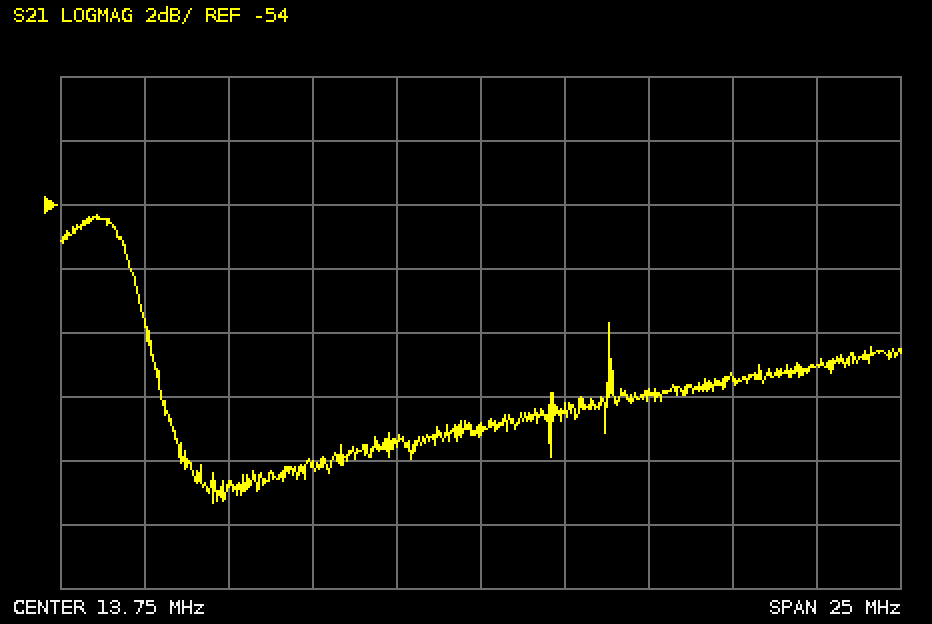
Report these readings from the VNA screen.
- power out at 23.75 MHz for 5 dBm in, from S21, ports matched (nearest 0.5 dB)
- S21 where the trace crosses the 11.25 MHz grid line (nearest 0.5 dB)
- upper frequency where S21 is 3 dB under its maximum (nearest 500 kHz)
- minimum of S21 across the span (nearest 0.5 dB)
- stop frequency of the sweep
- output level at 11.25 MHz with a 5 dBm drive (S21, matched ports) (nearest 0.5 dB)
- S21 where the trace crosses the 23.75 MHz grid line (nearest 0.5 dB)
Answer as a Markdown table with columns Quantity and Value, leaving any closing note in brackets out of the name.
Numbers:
| Quantity | Value |
|---|---|
| power out at 23.75 MHz for 5 dBm in, from S21, ports matched | -54.0 dBm |
| S21 where the trace crosses the 11.25 MHz grid line | -61.5 dB |
| upper frequency where S21 is 3 dB under its maximum | 3.5 MHz |
| minimum of S21 across the span | -63.5 dB |
| stop frequency of the sweep | 26.25 MHz |
| output level at 11.25 MHz with a 5 dBm drive (S21, matched ports) | -56.5 dBm |
| S21 where the trace crosses the 23.75 MHz grid line | -59.0 dB |
